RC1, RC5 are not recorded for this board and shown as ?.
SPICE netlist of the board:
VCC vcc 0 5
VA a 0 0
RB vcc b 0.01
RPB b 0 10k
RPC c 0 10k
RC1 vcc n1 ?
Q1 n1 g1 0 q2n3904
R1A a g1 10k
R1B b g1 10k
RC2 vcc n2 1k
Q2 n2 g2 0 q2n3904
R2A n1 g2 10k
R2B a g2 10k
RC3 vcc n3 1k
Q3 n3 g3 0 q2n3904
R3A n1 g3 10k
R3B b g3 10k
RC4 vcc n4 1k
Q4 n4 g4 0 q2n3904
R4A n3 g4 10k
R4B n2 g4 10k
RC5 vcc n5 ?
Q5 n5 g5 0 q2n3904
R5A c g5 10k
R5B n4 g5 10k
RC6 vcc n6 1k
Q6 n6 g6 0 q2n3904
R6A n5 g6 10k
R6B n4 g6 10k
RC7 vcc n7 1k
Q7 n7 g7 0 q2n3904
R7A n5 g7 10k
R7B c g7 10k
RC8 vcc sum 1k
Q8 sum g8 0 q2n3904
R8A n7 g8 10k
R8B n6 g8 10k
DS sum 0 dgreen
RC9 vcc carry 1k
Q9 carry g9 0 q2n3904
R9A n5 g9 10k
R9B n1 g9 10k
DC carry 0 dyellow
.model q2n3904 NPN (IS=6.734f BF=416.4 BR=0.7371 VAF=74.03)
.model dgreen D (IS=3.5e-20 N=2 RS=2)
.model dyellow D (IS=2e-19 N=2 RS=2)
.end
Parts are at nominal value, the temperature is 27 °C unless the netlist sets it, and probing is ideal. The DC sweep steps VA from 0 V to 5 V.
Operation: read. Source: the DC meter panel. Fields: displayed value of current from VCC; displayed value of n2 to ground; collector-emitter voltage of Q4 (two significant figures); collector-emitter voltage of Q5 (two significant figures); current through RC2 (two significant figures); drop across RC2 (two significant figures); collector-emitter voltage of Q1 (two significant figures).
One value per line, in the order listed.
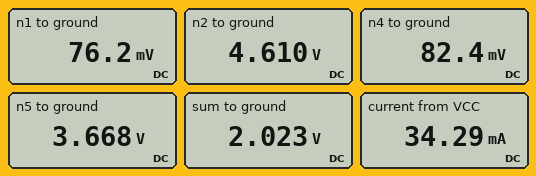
34.29 mA
4.610 V
82 mV
3.7 V
390 µA
390 mV
76 mV
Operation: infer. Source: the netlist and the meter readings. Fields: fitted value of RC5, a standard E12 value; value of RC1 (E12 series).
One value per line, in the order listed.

1.5 kΩ
1.2 kΩ
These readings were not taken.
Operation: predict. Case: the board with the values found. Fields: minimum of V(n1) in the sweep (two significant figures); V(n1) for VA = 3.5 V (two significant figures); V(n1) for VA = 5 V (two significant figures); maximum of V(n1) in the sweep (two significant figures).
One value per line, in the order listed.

58 mV
61 mV
58 mV
76 mV
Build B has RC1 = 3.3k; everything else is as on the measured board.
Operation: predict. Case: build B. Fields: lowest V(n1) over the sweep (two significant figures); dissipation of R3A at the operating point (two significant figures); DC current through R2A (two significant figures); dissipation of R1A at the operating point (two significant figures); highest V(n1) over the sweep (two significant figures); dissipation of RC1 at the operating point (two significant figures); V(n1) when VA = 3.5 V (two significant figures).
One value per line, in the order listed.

42 mV
43 µW
2.8 µA
47 µW
56 mV
7.4 mW
44 mV
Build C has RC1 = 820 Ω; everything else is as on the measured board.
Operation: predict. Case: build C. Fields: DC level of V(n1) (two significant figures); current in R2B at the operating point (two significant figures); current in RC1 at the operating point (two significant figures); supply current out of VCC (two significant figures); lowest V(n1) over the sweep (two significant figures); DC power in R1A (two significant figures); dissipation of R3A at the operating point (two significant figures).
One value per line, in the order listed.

85 mV
4.3 µA
6.0 mA
36 mA
65 mV
51 µW
39 µW
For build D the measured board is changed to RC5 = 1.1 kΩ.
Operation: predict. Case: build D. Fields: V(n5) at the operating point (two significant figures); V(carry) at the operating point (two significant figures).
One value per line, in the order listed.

3.9 V
88 mV
